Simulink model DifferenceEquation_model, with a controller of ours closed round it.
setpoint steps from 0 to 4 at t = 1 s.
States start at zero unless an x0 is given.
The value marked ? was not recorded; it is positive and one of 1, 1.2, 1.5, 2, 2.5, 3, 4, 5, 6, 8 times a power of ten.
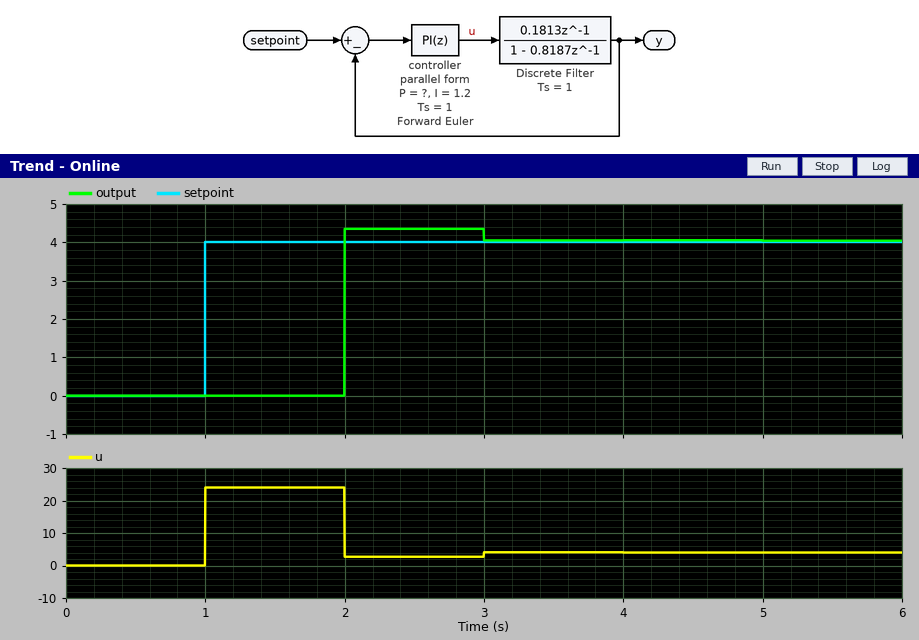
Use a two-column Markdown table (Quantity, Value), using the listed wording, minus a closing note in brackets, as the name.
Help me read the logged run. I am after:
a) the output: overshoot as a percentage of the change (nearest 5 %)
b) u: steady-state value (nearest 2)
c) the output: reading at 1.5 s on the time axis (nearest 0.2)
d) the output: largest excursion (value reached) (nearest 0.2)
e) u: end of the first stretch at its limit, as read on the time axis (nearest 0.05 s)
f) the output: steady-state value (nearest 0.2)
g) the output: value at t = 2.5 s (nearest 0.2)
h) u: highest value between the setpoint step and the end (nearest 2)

| Quantity | Value |
|---|---|
| the output: overshoot as a percentage of the change | 10 % |
| u: steady-state value | 4 |
| the output: reading at 1.5 s on the time axis | 0.0 |
| the output: largest excursion (value reached) | 4.4 |
| u: end of the first stretch at its limit, as read on the time axis | 2.00 s |
| the output: steady-state value | 4.0 |
| the output: value at t = 2.5 s | 4.4 |
| u: highest value between the setpoint step and the end | 24 |
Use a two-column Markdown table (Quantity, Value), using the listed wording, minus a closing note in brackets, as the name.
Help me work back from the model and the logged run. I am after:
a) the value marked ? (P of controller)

| Quantity | Value |
|---|---|
| the value marked ? | 6 |
